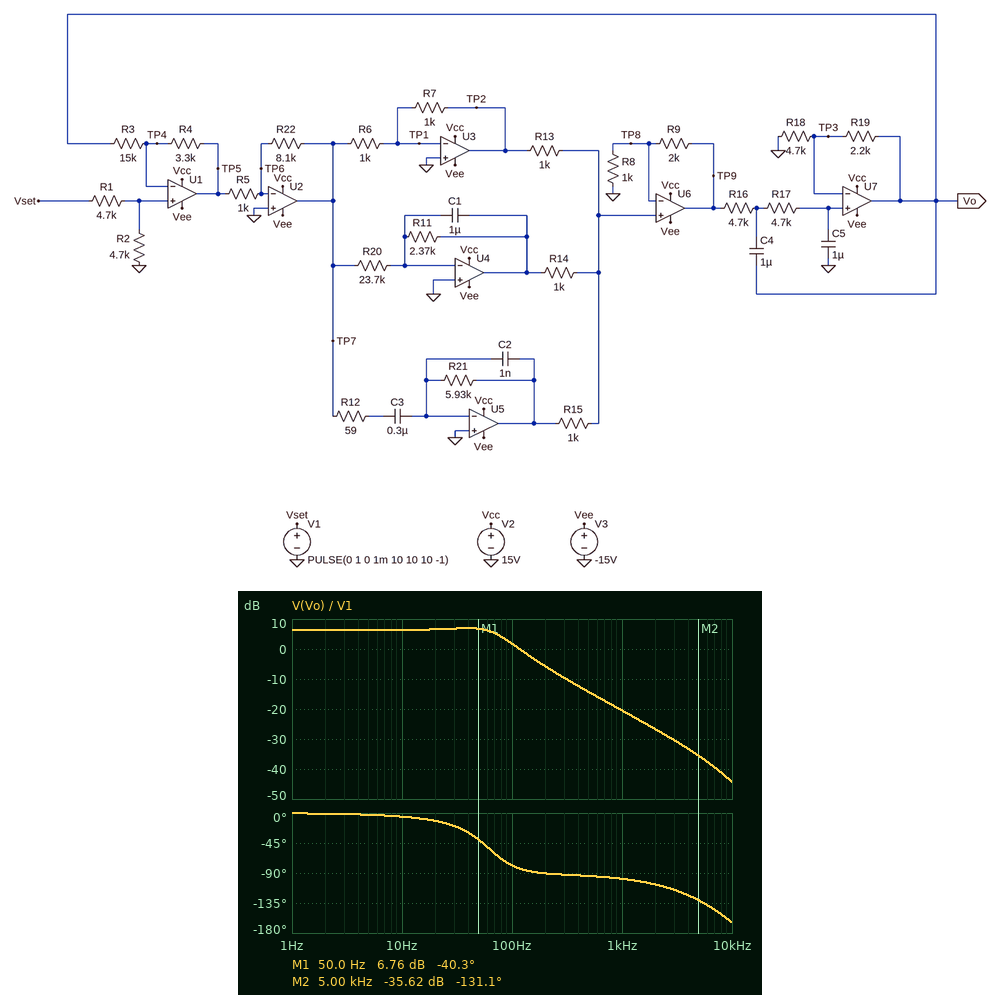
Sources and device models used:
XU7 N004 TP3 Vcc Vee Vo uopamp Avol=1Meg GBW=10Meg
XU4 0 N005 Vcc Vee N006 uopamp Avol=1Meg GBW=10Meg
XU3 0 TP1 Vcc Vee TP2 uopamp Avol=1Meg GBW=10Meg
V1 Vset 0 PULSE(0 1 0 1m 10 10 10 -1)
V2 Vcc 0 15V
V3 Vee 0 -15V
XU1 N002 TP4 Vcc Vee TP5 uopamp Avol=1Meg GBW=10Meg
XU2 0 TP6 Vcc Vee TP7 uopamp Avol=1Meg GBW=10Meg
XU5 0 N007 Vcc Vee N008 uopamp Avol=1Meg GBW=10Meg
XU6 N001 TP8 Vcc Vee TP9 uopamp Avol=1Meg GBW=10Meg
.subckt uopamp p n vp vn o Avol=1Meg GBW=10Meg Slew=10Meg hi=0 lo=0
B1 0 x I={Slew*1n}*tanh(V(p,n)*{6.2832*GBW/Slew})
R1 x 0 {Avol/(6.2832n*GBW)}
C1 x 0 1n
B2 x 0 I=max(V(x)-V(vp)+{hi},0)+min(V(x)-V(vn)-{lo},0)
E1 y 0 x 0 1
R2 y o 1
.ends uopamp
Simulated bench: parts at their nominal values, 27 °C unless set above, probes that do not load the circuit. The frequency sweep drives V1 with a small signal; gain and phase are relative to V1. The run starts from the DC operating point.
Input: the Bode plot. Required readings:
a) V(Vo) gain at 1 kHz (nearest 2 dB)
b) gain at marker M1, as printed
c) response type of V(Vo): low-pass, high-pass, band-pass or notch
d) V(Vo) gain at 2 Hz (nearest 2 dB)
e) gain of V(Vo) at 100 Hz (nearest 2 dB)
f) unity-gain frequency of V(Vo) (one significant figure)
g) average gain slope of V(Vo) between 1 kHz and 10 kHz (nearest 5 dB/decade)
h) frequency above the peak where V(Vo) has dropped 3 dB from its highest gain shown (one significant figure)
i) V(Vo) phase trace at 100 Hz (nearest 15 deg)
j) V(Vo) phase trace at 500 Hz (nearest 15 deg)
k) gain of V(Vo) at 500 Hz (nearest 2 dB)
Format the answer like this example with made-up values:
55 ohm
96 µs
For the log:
-20 dB
6.76 dB
low-pass
6 dB
2 dB
100 Hz
-25 dB/decade
80 Hz
-75 deg
-90 deg
-14 dB
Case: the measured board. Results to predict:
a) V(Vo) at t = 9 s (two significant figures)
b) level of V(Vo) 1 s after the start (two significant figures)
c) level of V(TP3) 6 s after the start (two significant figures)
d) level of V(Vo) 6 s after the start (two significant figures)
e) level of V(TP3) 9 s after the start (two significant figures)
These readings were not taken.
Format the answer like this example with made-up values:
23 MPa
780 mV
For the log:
2.1 V
2.1 V
1.4 V
2.1 V
1.4 V
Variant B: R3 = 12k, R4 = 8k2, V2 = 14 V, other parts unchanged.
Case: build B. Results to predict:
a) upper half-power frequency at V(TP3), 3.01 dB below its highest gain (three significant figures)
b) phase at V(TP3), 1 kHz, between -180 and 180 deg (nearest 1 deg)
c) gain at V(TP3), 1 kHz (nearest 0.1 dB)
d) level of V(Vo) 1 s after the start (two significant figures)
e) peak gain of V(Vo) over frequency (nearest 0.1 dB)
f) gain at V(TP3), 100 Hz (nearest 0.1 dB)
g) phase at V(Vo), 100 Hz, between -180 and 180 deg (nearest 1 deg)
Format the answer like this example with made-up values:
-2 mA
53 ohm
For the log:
151 Hz
-95 deg
-21.0 dB
1.1 V
1.7 dB
-2.3 dB
-41 deg
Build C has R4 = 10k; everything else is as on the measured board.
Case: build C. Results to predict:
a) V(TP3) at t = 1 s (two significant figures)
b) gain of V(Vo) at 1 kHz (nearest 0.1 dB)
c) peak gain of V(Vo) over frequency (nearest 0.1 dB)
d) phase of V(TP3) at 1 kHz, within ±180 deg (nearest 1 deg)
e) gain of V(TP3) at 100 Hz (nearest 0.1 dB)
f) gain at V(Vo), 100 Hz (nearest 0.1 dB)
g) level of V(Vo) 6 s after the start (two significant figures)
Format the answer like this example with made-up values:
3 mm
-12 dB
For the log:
760 mV
-17.7 dB
1.8 dB
-95 deg
-2.2 dB
1.1 dB
1.1 V
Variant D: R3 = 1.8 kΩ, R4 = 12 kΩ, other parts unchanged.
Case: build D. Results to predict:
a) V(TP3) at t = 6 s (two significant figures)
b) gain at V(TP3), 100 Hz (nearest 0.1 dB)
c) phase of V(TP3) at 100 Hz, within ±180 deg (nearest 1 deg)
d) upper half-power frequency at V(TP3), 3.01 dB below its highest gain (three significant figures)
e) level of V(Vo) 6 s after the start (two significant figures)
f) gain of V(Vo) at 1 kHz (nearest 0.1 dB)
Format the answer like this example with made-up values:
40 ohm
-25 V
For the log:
390 mV
-8.0 dB
-4 deg
1.22 kHz
570 mV
-6.8 dB
